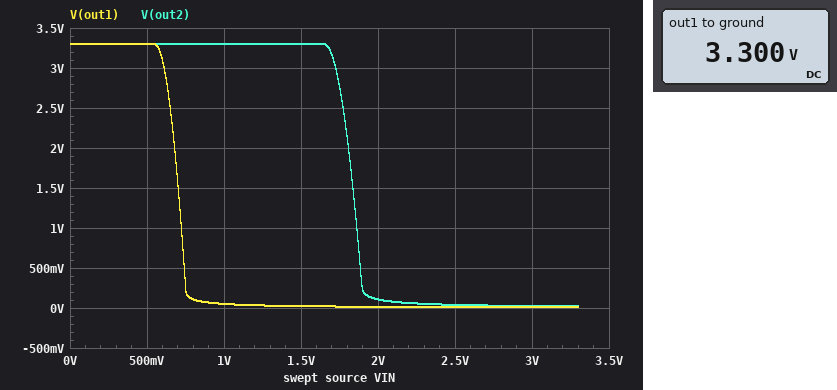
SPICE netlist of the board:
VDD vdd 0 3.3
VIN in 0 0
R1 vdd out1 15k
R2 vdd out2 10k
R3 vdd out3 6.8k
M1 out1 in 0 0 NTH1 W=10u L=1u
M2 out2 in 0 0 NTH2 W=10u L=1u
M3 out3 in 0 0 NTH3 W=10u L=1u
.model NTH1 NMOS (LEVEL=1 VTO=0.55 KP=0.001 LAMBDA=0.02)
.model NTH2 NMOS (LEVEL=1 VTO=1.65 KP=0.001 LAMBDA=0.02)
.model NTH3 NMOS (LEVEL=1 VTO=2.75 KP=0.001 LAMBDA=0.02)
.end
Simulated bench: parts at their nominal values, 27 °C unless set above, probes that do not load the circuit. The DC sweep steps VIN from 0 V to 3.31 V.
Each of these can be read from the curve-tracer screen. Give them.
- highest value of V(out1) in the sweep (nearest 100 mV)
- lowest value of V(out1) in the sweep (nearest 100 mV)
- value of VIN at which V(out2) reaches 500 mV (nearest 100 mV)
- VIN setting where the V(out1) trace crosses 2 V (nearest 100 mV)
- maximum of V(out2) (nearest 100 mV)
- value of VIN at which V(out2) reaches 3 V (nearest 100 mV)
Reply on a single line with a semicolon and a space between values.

3.3 V; 0 V; 1.9 V; 700 mV; 3.3 V; 1.7 V
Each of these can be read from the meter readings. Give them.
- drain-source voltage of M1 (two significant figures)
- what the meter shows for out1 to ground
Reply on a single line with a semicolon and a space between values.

3.3 V; 3.300 V
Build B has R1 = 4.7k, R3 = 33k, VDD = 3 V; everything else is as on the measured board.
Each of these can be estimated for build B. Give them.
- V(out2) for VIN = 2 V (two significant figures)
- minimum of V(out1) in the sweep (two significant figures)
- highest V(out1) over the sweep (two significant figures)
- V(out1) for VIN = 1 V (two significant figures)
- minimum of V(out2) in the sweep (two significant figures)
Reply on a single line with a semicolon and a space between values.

96 mV; 23 mV; 3.0 V; 160 mV; 18 mV
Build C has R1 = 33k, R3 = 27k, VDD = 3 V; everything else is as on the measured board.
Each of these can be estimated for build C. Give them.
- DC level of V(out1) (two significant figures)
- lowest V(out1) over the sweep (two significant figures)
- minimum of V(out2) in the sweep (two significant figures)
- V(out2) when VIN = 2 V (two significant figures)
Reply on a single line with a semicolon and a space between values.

3.0 V; 3.3 mV; 18 mV; 96 mV
